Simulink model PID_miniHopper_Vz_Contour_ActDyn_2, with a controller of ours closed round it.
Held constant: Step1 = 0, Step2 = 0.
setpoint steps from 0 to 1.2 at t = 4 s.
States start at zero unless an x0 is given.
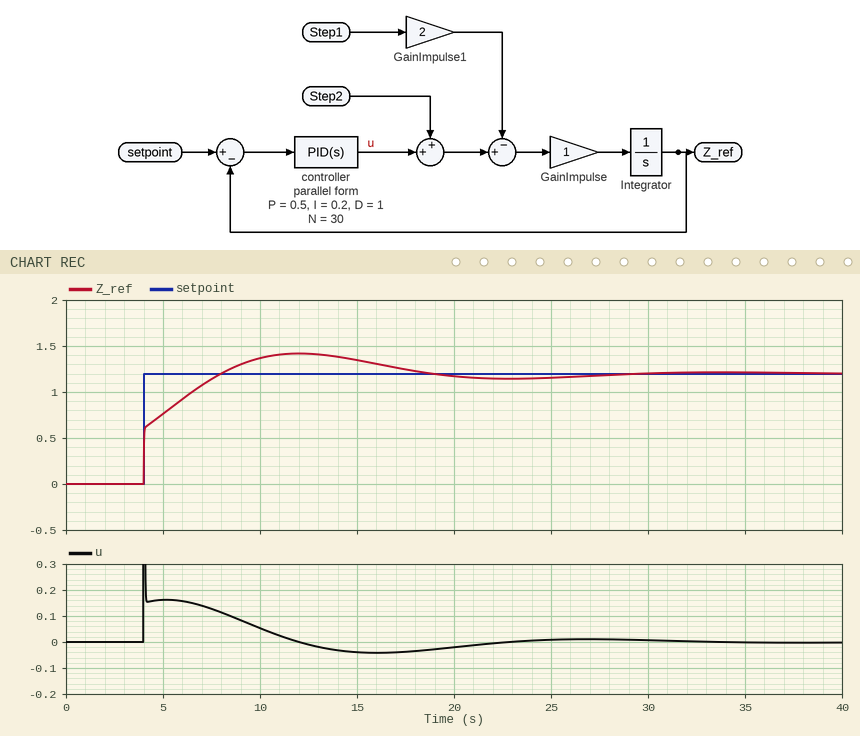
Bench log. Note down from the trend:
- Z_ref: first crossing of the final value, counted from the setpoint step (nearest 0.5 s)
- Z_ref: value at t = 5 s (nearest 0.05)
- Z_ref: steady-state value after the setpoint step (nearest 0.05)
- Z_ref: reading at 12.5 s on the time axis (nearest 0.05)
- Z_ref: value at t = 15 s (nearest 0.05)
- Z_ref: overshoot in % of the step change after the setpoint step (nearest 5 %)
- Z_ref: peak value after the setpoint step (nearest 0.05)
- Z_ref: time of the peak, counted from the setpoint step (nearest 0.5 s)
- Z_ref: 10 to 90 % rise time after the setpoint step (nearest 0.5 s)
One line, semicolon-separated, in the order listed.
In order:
4.0 s; 0.75; 1.20; 1.40; 1.35; 20 %; 1.40; 8.0 s; 3.0 s
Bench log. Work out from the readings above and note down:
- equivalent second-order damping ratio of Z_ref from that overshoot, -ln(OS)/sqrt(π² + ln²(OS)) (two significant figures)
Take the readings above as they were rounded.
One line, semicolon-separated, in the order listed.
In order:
0.46
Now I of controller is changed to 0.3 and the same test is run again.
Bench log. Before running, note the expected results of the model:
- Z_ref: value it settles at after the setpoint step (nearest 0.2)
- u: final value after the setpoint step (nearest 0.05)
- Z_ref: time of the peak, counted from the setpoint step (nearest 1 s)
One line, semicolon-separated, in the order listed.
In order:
1.2; 0.00; 7 s
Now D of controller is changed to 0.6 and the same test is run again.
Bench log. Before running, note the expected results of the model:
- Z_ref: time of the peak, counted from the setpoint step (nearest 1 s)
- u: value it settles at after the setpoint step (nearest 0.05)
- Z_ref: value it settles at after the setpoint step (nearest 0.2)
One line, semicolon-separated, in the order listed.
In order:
7 s; 0.00; 1.2
